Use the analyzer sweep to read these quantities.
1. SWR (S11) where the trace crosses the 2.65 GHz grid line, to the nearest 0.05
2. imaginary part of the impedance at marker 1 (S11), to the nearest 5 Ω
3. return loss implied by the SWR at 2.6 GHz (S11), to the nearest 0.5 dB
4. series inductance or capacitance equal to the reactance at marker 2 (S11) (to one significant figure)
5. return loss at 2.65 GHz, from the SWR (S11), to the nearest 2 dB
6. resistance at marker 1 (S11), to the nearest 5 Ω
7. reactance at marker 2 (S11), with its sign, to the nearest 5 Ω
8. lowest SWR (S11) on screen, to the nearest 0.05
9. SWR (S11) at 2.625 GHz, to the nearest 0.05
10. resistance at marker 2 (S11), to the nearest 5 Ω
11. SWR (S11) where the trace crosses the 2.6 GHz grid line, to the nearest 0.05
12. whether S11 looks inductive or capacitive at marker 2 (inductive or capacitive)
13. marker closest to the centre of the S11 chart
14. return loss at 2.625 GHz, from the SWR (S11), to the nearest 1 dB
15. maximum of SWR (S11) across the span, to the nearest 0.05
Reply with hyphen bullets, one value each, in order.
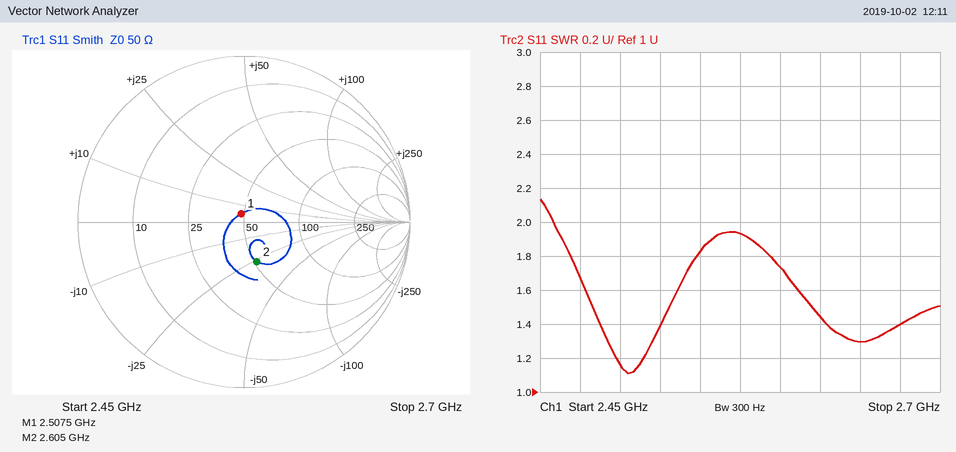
- 1.30
- +5 Ω
- 11.5 dB
- 2 pF
- 18 dB
- 50 Ω
- -25 Ω
- 1.10
- 1.45
- 50 Ω
- 1.75
- capacitive
- marker 1
- 15 dB
- 2.15
